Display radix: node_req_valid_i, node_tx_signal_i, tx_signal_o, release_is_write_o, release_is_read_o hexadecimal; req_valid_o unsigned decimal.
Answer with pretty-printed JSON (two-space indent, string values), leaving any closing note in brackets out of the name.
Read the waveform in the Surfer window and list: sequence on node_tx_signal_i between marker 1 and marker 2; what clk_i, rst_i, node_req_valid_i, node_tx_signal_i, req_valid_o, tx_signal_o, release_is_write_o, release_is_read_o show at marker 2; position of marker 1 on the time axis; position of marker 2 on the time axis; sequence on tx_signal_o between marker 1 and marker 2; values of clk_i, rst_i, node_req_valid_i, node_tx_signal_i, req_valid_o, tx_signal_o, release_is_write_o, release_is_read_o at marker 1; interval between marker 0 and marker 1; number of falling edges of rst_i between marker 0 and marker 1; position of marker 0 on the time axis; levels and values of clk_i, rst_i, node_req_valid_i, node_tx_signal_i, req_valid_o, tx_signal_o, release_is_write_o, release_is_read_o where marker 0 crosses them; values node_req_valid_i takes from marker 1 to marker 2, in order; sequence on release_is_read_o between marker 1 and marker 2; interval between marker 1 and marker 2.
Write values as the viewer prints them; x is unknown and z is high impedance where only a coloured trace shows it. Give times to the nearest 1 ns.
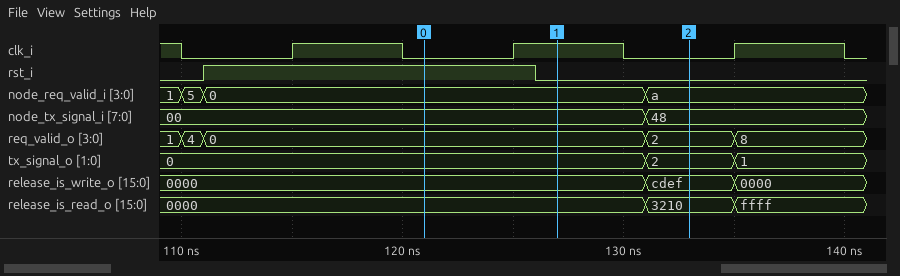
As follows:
{
  "sequence on node_tx_signal_i between marker 1 and marker 2": "00, 48",
  "what clk_i, rst_i, node_req_valid_i, node_tx_signal_i, req_valid_o, tx_signal_o, release_is_write_o, release_is_read_o show at marker 2": "clk_i=0, rst_i=0, node_req_valid_i=a, node_tx_signal_i=48, req_valid_o=2, tx_signal_o=2, release_is_write_o=cdef, release_is_read_o=3210",
  "position of marker 1 on the time axis": "127 ns",
  "position of marker 2 on the time axis": "133 ns",
  "sequence on tx_signal_o between marker 1 and marker 2": "0, 2",
  "values of clk_i, rst_i, node_req_valid_i, node_tx_signal_i, req_valid_o, tx_signal_o, release_is_write_o, release_is_read_o at marker 1": "clk_i=1, rst_i=0, node_req_valid_i=0, node_tx_signal_i=00, req_valid_o=0, tx_signal_o=0, release_is_write_o=0000, release_is_read_o=0000",
  "interval between marker 0 and marker 1": "6 ns",
  "number of falling edges of rst_i between marker 0 and marker 1": "1",
  "position of marker 0 on the time axis": "121 ns",
  "levels and values of clk_i, rst_i, node_req_valid_i, node_tx_signal_i, req_valid_o, tx_signal_o, release_is_write_o, release_is_read_o where marker 0 crosses them": "clk_i=0, rst_i=1, node_req_valid_i=0, node_tx_signal_i=00, req_valid_o=0, tx_signal_o=0, release_is_write_o=0000, release_is_read_o=0000",
  "values node_req_valid_i takes from marker 1 to marker 2, in order": "0, a",
  "sequence on release_is_read_o between marker 1 and marker 2": "0000, 3210",
  "interval between marker 1 and marker 2": "6 ns"
}
